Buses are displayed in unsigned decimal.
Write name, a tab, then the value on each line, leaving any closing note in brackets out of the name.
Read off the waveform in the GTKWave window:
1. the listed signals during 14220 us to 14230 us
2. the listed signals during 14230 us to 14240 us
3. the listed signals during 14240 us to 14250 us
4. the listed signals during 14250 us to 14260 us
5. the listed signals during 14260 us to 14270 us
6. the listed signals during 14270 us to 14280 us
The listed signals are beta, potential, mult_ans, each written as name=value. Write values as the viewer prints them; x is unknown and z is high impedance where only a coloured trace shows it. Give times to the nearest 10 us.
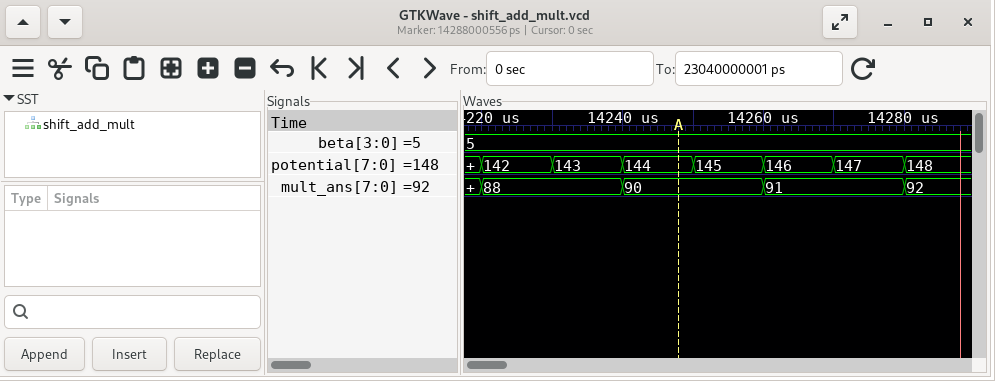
the listed signals during 14220 us to 14230 us	beta=5, potential=142, mult_ans=88
the listed signals during 14230 us to 14240 us	beta=5, potential=143, mult_ans=88
the listed signals during 14240 us to 14250 us	beta=5, potential=144, mult_ans=90
the listed signals during 14250 us to 14260 us	beta=5, potential=145, mult_ans=90
the listed signals during 14260 us to 14270 us	beta=5, potential=146, mult_ans=91
the listed signals during 14270 us to 14280 us	beta=5, potential=147, mult_ans=91
